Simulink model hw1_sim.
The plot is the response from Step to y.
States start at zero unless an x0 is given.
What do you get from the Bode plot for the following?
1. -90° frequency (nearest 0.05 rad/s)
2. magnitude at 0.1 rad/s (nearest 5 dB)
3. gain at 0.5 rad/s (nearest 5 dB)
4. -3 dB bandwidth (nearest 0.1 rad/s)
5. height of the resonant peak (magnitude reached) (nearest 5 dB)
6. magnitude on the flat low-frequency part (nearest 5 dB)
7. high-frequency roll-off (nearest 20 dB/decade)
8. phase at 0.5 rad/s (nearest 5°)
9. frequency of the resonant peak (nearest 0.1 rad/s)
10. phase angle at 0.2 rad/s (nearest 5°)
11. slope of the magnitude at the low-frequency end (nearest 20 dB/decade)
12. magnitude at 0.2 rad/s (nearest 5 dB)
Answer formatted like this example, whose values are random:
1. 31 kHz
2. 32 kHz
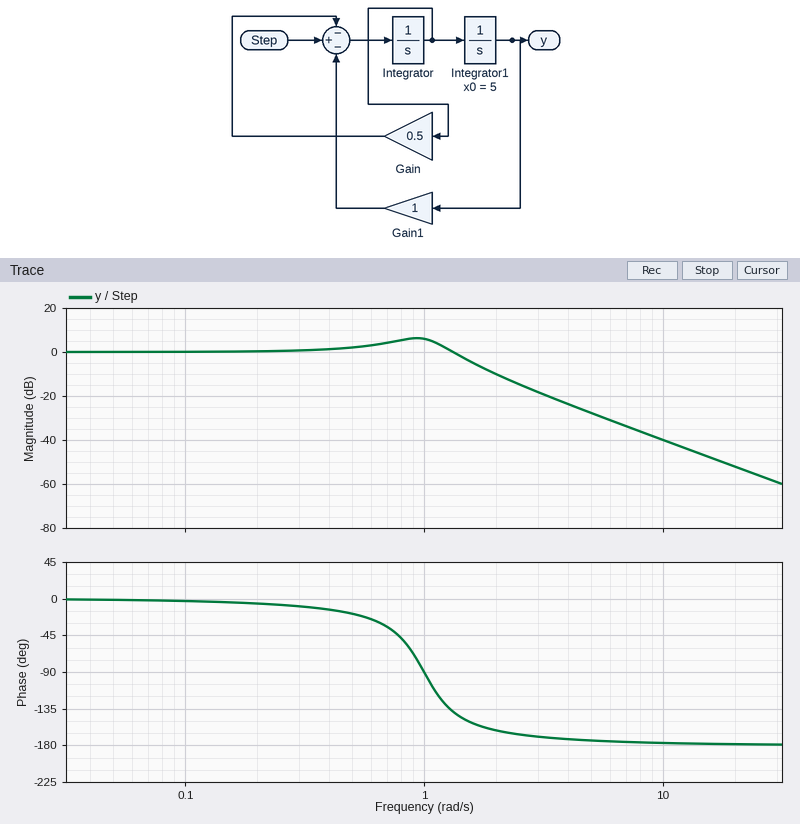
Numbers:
1. 1.00 rad/s
2. 0 dB
3. 0 dB
4. 1.5 rad/s
5. 5 dB
6. 0 dB
7. -40 dB/decade
8. -20°
9. 0.9 rad/s
10. -5°
11. 0 dB/decade
12. 0 dB
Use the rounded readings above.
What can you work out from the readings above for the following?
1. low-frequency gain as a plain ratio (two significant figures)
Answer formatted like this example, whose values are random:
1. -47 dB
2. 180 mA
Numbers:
1. 1.0
